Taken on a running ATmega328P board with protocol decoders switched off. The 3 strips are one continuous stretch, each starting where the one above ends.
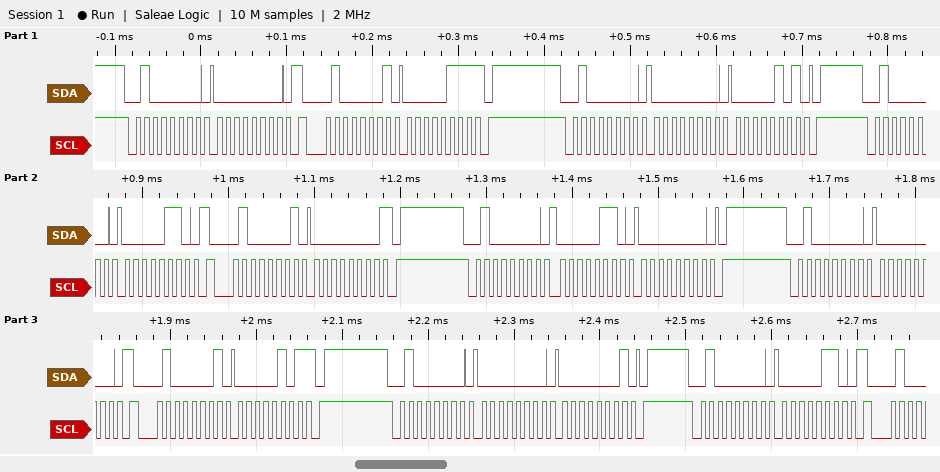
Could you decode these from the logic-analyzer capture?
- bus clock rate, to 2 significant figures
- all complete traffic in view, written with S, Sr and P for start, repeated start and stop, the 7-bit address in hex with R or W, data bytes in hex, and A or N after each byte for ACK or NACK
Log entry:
100 kHz
S 20W A 00 A Sr 20R A 07 N P S 20W A 00 A 05 A P S 20W A 06 A Sr 20R A 00 N P S 20W A 06 A 00 A P S 20W A 00 A Sr 20R A 05 N P S 20W A 00 A 01 A P S 20W A 06 A
